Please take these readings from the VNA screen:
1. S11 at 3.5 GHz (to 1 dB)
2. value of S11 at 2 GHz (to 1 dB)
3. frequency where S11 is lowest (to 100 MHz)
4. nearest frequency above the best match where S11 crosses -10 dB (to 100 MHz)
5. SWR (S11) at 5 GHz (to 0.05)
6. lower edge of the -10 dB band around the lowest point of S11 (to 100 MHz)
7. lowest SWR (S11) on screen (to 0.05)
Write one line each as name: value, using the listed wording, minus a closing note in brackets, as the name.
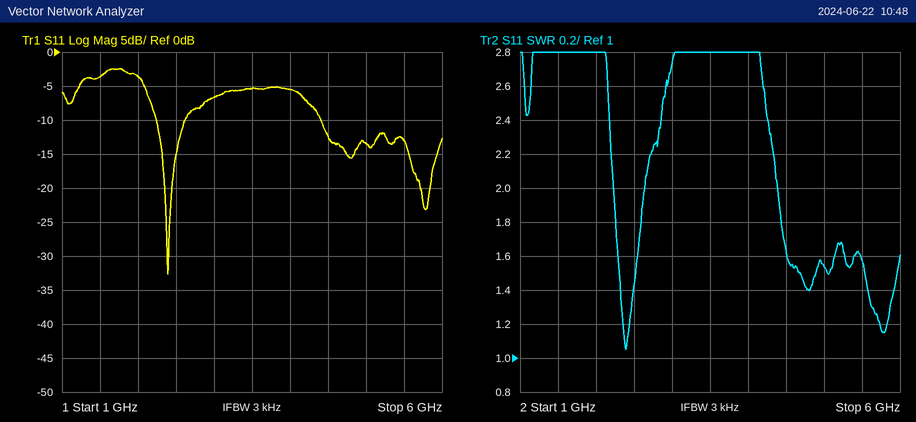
S11 at 3.5 GHz: -5 dB
value of S11 at 2 GHz: -4 dB
frequency where S11 is lowest: 2.4 GHz
nearest frequency above the best match where S11 crosses -10 dB: 2.6 GHz
SWR (S11) at 5 GHz: 1.55
lower edge of the -10 dB band around the lowest point of S11: 2.2 GHz
lowest SWR (S11) on screen: 1.05
